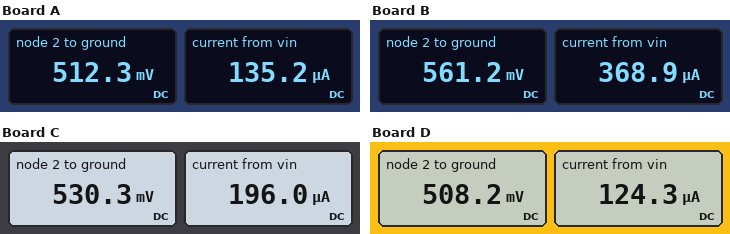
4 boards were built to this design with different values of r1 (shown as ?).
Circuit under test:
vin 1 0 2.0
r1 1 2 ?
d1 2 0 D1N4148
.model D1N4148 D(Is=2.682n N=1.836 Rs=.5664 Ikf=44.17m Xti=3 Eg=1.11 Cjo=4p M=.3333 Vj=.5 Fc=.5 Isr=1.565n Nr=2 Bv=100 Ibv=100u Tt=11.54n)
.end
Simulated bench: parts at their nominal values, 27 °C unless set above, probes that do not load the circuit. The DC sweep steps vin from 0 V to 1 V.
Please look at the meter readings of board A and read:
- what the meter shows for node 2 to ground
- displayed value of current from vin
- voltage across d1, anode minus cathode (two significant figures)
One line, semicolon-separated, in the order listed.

512.3 mV; 135.2 µA; 510 mV
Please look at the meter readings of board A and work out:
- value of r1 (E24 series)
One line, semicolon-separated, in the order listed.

11 kΩ
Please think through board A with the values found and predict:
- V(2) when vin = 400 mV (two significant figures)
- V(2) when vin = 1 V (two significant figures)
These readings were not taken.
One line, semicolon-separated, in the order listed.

350 mV; 460 mV
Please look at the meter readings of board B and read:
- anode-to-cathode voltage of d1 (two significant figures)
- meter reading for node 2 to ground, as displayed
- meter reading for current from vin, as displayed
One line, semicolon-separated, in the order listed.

560 mV; 561.2 mV; 368.9 µA
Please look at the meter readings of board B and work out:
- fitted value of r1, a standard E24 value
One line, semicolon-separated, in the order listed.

3.9 kΩ
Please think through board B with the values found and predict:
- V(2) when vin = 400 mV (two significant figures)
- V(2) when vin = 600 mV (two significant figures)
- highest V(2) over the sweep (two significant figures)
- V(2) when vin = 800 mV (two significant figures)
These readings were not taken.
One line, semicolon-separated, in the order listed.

370 mV; 450 mV; 510 mV; 490 mV
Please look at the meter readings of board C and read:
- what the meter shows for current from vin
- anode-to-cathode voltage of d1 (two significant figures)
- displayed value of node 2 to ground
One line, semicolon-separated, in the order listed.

196.0 µA; 530 mV; 530.3 mV
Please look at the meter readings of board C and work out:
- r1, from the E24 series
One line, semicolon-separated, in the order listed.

7.5 kΩ
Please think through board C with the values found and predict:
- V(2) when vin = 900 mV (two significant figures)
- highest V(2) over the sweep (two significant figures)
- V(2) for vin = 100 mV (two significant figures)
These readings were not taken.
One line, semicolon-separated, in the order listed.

470 mV; 480 mV; 100 mV
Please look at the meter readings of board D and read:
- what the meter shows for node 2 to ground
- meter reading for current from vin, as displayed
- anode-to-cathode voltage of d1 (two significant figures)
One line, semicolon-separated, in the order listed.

508.2 mV; 124.3 µA; 510 mV
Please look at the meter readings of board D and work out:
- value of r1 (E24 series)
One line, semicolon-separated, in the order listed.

12 kΩ
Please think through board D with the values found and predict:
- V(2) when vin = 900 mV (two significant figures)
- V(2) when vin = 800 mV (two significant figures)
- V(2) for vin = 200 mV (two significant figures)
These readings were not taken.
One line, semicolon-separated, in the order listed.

450 mV; 440 mV; 200 mV
